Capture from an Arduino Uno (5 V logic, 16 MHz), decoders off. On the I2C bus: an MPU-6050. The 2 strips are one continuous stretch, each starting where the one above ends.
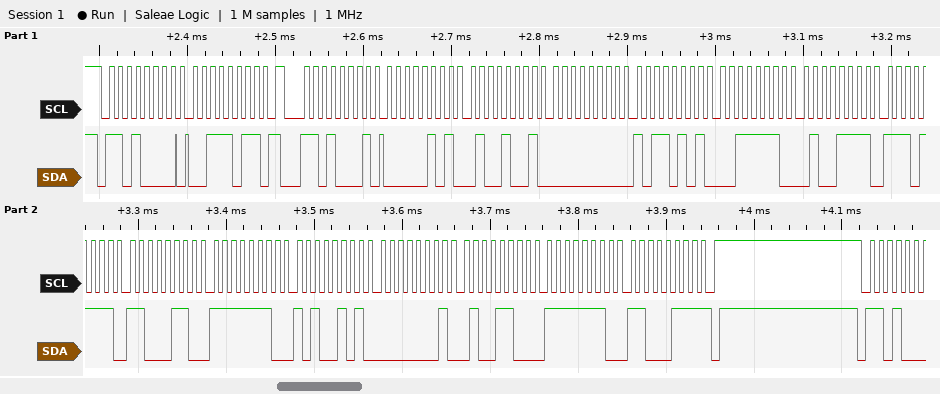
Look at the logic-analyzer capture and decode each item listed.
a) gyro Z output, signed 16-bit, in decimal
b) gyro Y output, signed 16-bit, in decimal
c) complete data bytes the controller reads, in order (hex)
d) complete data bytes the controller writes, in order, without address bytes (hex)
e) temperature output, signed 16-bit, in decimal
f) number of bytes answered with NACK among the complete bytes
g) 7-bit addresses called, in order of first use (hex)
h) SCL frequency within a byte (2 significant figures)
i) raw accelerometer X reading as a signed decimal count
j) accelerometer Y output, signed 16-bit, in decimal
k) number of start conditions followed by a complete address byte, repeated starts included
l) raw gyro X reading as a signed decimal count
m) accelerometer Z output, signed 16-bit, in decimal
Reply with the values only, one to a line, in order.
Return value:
-313
332
05 49 00 B5 3E 4F EF C6 FE A5 01 4C FE C7
3B
-4154
1
0x68
100 kHz
1353
181
2
-347
15951
